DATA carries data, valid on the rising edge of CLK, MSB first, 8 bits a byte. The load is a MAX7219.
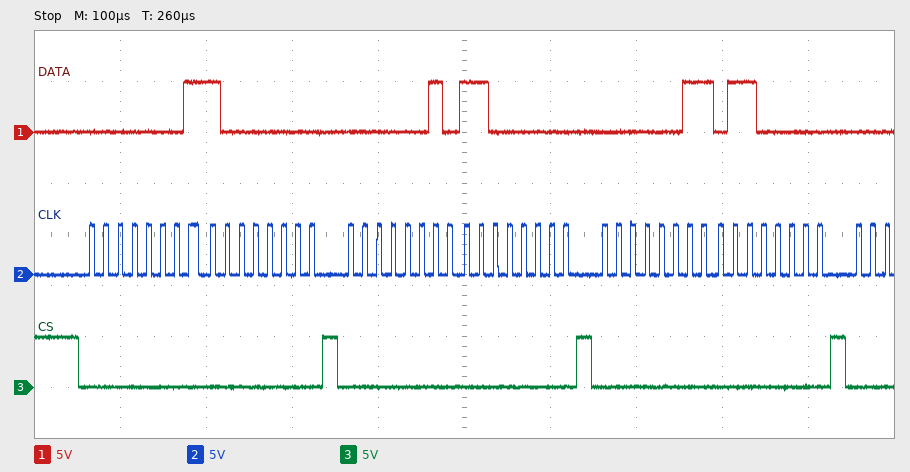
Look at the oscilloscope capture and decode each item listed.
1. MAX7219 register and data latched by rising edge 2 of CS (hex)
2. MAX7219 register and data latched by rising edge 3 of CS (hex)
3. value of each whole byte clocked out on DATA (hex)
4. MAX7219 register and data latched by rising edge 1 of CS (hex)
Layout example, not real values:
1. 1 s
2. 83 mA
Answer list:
1. register 0x2, data 0xC0
2. register 0x3, data 0x60
3. 01 80 02 C0 03 60
4. register 0x1, data 0x80
